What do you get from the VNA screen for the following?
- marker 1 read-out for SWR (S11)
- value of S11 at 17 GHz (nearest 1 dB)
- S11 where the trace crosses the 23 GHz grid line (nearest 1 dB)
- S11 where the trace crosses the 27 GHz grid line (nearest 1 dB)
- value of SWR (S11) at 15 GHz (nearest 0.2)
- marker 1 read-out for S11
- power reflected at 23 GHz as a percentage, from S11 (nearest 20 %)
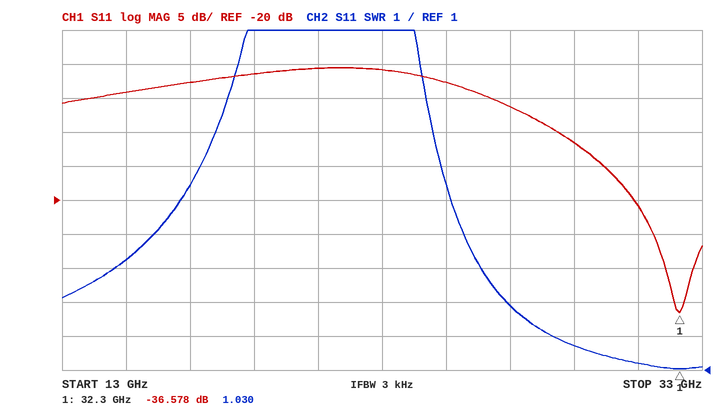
1.030
-3 dB
-1 dB
-6 dB
4.2
-36.578 dB
80 %
